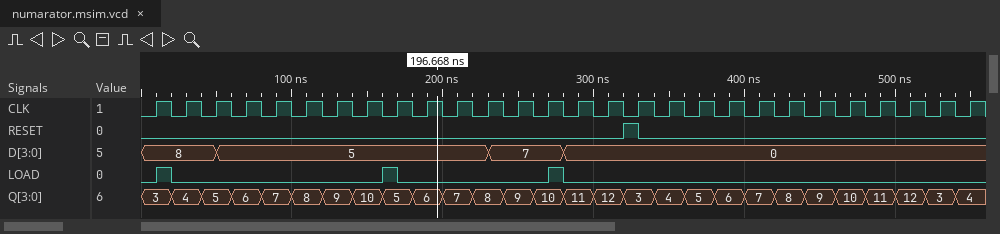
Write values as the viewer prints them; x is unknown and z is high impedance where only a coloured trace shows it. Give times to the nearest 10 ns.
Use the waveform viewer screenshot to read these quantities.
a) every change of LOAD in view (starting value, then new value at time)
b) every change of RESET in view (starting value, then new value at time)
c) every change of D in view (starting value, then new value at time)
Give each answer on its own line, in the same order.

0, 1 at 10 ns, 0 at 20 ns, 1 at 160 ns, 0 at 170 ns, 1 at 270 ns, 0 at 280 ns
0, 1 at 320 ns, 0 at 330 ns
8, 5 at 50 ns, 7 at 230 ns, 0 at 280 ns
